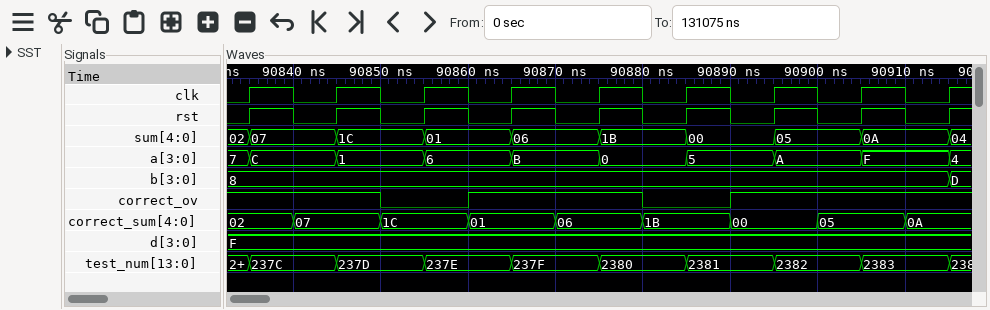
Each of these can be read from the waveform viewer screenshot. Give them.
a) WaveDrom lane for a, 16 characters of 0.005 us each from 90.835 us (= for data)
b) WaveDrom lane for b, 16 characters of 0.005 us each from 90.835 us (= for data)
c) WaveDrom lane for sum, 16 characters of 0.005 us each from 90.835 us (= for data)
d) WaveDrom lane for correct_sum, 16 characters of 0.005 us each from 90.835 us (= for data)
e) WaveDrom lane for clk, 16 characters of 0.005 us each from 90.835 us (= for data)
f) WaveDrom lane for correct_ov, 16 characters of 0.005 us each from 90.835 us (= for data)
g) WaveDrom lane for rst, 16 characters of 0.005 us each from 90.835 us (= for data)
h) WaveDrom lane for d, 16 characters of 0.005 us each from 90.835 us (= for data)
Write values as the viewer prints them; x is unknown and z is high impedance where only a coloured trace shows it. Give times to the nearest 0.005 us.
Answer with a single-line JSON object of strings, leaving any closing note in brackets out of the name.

{"WaveDrom lane for a, 16 characters of 0.005 us each from 90.835 us": "{name: 'a', wave: '=.=.=.=.=.=.=.=.', data: 'C 1 6 B 0 5 A F'}", "WaveDrom lane for b, 16 characters of 0.005 us each from 90.835 us": "{name: 'b', wave: '=...............', data: '8'}", "WaveDrom lane for sum, 16 characters of 0.005 us each from 90.835 us": "{name: 'sum', wave: '=.=.=.=.=.=.=.=.', data: '07 1C 01 06 1B 00 05 0A'}", "WaveDrom lane for correct_sum, 16 characters of 0.005 us each from 90.835 us": "{name: 'correct_sum', wave: '==.=.=.=.=.=.=.=', data: '02 07 1C 01 06 1B 00 05 0A'}", "WaveDrom lane for clk, 16 characters of 0.005 us each from 90.835 us": "{name: 'clk', wave: '1010101010101010'}", "WaveDrom lane for correct_ov, 16 characters of 0.005 us each from 90.835 us": "{name: 'correct_ov', wave: '1..0.1...0.1....'}", "WaveDrom lane for rst, 16 characters of 0.005 us each from 90.835 us": "{name: 'rst', wave: '1010101010101010'}", "WaveDrom lane for d, 16 characters of 0.005 us each from 90.835 us": "{name: 'd', wave: '=...............', data: 'F'}"}
